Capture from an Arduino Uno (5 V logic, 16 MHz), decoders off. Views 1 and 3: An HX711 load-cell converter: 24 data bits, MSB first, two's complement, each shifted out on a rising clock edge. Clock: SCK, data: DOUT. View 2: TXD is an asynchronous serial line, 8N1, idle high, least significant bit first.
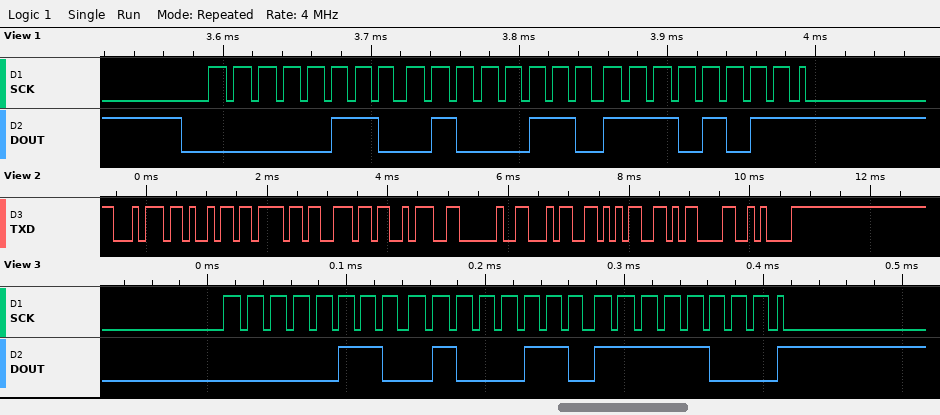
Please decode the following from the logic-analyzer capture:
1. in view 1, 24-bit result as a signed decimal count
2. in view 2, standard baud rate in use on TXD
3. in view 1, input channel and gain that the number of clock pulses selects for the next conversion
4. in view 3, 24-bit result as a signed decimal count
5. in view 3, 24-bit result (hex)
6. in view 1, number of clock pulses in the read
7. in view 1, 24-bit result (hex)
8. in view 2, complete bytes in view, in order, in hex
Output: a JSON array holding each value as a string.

["411371", "9600 baud", "channel A, gain 128", "411384", "0x0646F8", "25", "0x0646EB", "74 69 6F 6E 3A 20 34 35 0D 0A"]
